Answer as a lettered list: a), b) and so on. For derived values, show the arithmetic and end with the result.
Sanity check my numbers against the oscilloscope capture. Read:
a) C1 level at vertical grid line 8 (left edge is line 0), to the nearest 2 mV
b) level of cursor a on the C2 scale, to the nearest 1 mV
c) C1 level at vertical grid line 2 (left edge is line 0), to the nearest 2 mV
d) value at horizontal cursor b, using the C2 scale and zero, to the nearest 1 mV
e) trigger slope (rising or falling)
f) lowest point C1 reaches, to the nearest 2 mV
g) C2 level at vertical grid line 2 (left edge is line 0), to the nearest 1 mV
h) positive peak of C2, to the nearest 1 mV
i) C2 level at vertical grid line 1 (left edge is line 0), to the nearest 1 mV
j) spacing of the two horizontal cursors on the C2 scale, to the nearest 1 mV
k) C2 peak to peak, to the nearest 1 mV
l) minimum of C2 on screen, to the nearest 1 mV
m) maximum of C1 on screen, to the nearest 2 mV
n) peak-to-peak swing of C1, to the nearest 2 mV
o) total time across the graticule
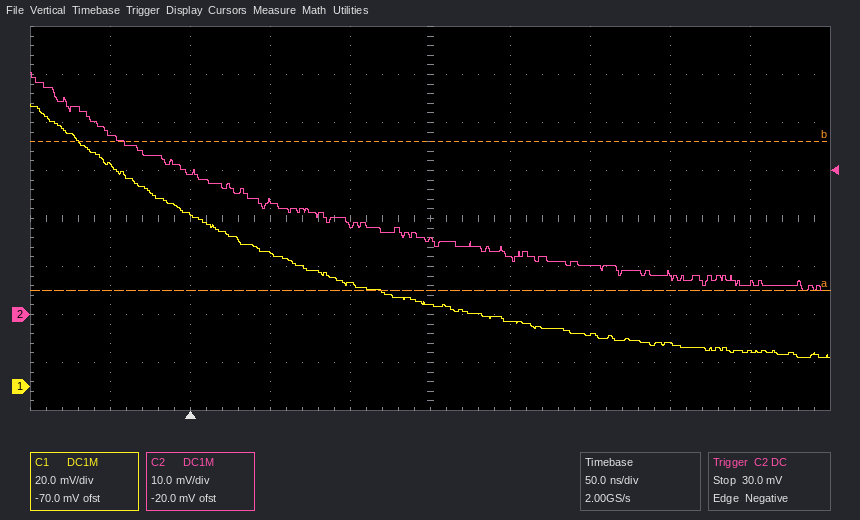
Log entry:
a) 18 mV
b) 5 mV
c) 72 mV
d) 36 mV
e) falling
f) 12 mV
g) 30 mV
h) 50 mV
i) 38 mV
j) 31 mV
k) 50 mV − (5 mV) = 45 mV
l) 5 mV
m) 118 mV
n) 118 mV − (12 mV) = 106 mV
o) 500 ns
